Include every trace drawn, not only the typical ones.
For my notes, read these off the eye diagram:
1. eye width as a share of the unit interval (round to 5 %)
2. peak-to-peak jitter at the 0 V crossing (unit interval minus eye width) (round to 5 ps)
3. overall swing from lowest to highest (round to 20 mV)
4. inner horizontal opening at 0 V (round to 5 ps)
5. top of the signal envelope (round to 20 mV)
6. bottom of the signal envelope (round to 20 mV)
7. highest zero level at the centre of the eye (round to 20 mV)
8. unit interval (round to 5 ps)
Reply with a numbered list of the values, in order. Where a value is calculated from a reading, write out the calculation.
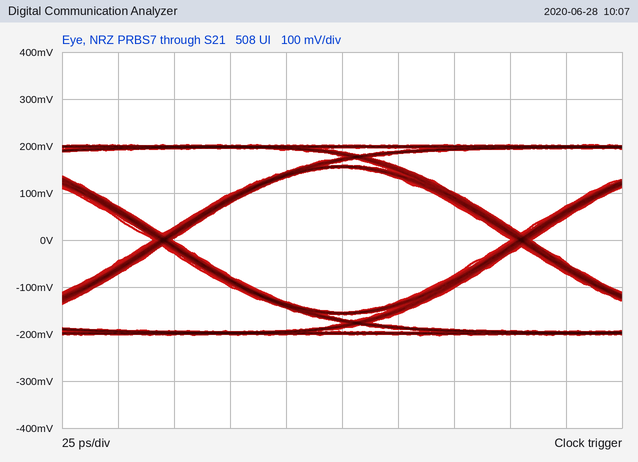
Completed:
1. 150 ps / 160 ps ≈ 93.8 %, so 95 % to the nearest 5 %
2. 10 ps
3. 400 mV
4. 150 ps
5. 200 mV
6. -200 mV
7. -160 mV
8. 160 ps
